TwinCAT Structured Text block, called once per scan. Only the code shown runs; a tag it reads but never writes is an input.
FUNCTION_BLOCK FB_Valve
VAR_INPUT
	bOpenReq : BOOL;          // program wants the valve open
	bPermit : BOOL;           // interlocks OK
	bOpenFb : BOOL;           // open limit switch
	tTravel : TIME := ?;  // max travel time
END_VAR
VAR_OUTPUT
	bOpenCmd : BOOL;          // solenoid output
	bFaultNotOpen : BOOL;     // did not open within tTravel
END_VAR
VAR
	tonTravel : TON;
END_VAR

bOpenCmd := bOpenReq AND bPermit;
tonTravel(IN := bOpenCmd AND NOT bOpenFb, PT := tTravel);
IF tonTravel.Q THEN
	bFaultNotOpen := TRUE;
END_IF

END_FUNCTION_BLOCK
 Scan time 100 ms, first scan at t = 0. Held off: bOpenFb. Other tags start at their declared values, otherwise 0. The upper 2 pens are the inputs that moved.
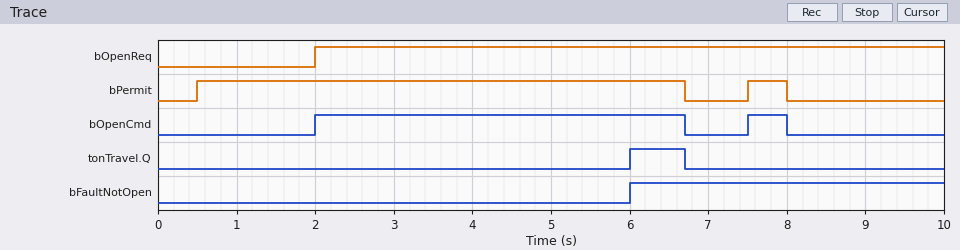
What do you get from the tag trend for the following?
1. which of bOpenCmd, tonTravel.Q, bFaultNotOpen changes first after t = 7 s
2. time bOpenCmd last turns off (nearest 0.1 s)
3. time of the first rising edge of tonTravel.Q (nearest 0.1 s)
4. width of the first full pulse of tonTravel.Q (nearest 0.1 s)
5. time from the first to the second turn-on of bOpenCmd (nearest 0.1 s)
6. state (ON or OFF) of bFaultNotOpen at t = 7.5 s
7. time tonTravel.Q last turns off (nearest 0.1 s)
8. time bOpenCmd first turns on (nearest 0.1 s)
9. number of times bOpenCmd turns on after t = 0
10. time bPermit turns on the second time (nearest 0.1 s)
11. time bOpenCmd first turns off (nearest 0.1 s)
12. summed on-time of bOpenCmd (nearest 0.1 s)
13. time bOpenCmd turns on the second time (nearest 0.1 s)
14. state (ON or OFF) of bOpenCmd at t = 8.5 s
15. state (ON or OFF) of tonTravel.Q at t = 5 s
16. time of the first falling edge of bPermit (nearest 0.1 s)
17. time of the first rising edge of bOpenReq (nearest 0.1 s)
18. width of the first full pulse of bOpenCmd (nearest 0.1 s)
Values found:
bOpenCmd
8.0 s
6.0 s
0.7 s
5.5 s
ON
6.7 s
2.0 s
2
7.5 s
6.7 s
5.2 s
7.5 s
OFF
OFF
6.7 s
2.0 s
4.7 s
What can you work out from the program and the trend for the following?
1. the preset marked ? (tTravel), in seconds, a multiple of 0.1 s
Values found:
4.0 s
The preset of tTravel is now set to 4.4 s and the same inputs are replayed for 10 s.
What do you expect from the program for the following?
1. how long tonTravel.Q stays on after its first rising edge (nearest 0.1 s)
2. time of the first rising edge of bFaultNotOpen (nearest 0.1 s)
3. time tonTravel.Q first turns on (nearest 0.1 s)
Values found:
0.3 s
6.4 s
6.4 s
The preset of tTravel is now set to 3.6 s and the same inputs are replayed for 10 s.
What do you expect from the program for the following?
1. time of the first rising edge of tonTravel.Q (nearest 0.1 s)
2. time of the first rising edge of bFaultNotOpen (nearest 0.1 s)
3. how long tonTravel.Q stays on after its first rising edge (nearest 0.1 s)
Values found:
5.6 s
5.6 s
1.1 s
